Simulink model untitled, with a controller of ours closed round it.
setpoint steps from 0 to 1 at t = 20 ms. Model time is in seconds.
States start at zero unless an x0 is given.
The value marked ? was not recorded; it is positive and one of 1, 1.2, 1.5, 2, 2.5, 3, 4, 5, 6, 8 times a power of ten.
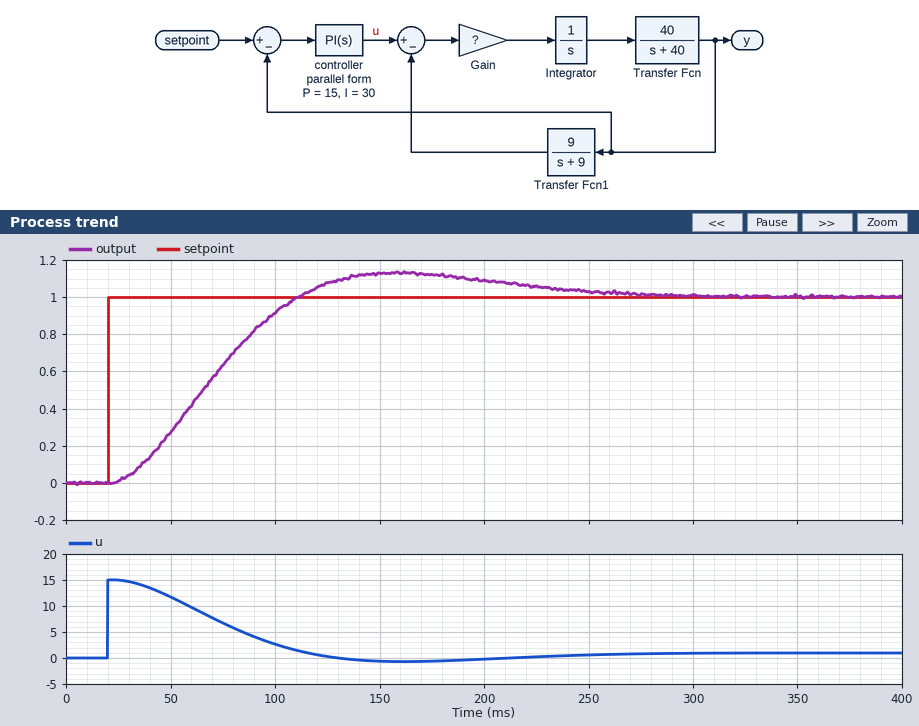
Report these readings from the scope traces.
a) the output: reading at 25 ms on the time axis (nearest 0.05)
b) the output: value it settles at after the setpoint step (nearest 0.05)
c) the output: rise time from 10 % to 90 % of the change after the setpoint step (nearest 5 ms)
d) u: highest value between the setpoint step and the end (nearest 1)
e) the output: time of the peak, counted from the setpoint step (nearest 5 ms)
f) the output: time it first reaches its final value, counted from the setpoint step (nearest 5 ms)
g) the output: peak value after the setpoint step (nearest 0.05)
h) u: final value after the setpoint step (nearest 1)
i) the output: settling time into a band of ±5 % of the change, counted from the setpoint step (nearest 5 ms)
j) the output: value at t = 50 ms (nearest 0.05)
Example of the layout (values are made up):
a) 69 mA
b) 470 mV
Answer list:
a) 0.00
b) 1.00
c) 60 ms
d) 15
e) 140 ms
f) 90 ms
g) 1.15
h) 1
i) 210 ms
j) 0.25
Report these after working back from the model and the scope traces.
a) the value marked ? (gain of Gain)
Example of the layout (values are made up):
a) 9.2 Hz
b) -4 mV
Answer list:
a) 1.5
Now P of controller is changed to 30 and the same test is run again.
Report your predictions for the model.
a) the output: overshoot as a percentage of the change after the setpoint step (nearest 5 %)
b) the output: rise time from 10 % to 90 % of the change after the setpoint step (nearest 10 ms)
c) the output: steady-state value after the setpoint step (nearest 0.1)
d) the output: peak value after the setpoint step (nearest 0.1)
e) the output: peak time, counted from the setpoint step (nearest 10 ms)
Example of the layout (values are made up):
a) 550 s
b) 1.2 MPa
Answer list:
a) 20 %
b) 40 ms
c) 1.0
d) 1.2
e) 80 ms
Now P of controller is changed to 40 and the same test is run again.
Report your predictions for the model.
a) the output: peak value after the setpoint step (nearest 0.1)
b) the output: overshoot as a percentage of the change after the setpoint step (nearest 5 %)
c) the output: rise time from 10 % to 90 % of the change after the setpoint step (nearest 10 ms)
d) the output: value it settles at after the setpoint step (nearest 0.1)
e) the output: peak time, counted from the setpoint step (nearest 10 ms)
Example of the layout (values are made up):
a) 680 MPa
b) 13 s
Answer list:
a) 1.3
b) 25 %
c) 30 ms
d) 1.0
e) 70 ms
